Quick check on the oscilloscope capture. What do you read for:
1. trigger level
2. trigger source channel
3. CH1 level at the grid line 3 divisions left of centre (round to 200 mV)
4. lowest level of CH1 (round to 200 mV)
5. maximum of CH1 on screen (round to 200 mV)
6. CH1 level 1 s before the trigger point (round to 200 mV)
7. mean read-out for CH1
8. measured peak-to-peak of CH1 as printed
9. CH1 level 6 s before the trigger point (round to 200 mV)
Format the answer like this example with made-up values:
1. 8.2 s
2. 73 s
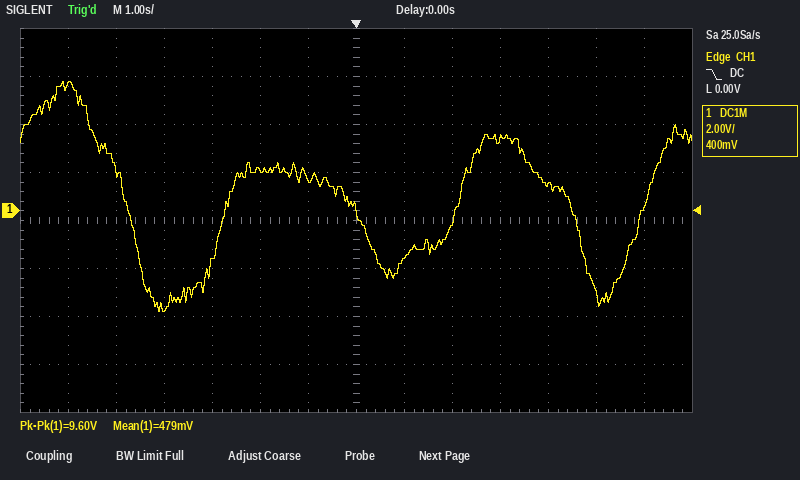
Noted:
1. 0.00 V
2. CH1
3. -2.2 V
4. -4.2 V
5. 5.4 V
6. 1.4 V
7. 479 mV
8. 9.60 V
9. 5.2 V
